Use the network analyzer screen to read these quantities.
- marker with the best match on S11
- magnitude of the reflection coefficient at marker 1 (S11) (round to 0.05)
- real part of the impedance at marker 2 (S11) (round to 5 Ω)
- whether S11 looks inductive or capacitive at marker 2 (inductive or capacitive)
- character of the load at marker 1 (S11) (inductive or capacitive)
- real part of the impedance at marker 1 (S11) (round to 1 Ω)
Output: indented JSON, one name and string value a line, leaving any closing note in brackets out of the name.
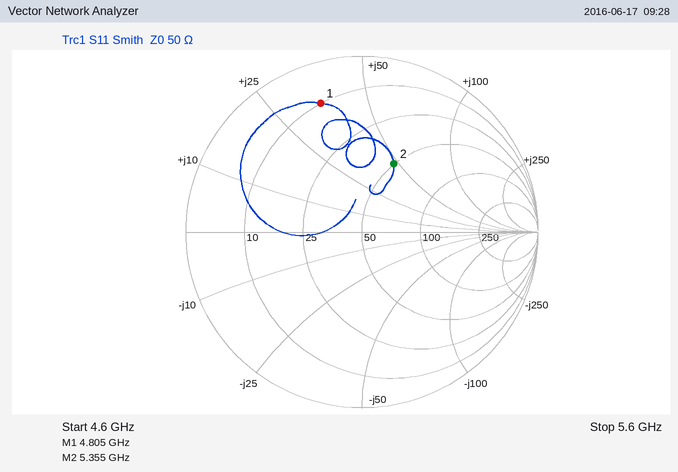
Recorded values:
{
  "marker with the best match on S11": "marker 2",
  "magnitude of the reflection coefficient at marker 1 (S11)": "0.75",
  "real part of the impedance at marker 2 (S11)": "50 Ω",
  "whether S11 looks inductive or capacitive at marker 2": "inductive",
  "character of the load at marker 1 (S11)": "inductive",
  "real part of the impedance at marker 1 (S11)": "10 Ω"
}
